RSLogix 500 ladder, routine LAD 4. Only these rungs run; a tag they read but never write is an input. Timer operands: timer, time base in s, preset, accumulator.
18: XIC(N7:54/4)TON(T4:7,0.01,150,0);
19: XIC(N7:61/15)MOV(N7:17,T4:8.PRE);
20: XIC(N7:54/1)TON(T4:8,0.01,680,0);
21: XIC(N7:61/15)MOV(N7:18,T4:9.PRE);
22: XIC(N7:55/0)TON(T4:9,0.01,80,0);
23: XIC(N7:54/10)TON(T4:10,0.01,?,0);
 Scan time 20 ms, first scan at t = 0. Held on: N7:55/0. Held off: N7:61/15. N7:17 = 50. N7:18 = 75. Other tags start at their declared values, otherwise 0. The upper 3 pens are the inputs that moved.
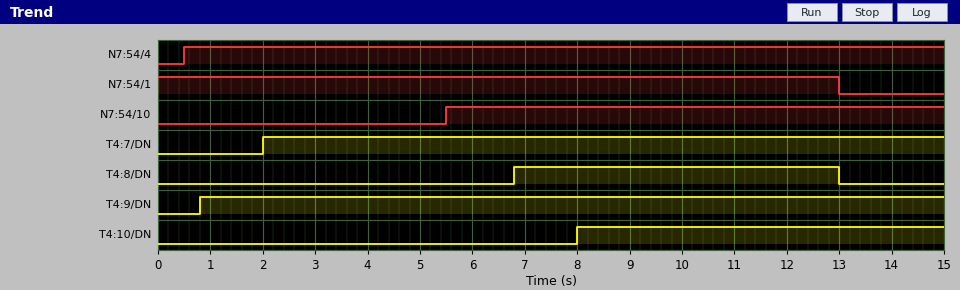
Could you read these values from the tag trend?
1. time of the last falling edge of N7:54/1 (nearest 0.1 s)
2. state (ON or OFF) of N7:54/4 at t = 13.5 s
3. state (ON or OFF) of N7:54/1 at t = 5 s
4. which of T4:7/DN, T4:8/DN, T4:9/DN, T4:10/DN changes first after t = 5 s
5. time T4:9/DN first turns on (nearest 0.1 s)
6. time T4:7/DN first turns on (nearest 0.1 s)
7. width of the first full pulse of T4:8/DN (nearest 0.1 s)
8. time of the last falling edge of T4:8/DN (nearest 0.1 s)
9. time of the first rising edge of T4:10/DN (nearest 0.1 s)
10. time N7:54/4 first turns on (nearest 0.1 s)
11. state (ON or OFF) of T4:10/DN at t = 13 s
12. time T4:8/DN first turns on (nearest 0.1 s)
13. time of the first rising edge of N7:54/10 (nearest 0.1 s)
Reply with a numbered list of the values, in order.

1. 13.0 s
2. ON
3. ON
4. T4:8/DN
5. 0.8 s
6. 2.0 s
7. 6.2 s
8. 13.0 s
9. 8.0 s
10. 0.5 s
11. ON
12. 6.8 s
13. 5.5 s
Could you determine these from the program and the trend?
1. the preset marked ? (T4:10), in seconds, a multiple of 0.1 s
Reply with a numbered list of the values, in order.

1. 2.5 s
